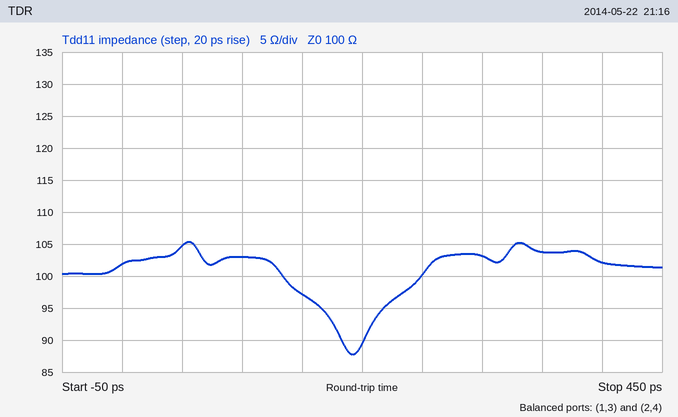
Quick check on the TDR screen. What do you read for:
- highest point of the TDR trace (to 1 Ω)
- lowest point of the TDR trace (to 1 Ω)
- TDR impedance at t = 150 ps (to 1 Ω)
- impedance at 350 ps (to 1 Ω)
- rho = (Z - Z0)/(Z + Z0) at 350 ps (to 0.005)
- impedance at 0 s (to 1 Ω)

105 Ω
88 Ω
97 Ω
104 Ω
+0.020
102 Ω
